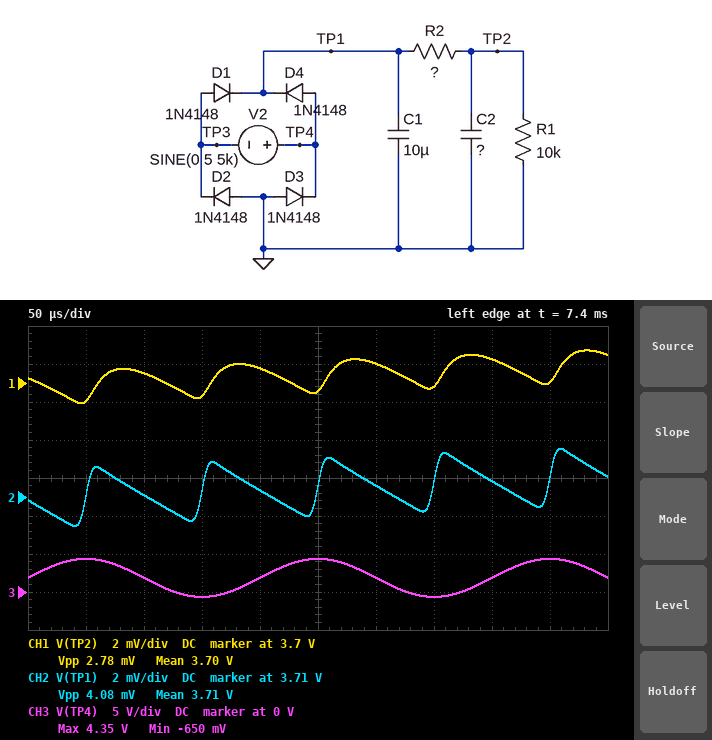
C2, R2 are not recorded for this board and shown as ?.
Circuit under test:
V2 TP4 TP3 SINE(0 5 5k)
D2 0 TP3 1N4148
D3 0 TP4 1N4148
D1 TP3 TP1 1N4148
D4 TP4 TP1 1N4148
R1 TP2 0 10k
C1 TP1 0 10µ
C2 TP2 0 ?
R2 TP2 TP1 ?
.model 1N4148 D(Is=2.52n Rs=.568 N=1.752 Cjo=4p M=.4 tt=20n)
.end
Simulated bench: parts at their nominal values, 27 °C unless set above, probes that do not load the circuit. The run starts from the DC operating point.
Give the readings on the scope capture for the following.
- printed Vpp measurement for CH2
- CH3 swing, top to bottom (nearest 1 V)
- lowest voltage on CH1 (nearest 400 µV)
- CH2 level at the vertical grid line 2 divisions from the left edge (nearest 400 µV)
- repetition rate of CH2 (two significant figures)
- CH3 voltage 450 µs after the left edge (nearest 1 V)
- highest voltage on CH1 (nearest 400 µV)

4.08 mV
5 V
3.6988 V
3.7100 V
10 kHz
4 V
3.7016 V
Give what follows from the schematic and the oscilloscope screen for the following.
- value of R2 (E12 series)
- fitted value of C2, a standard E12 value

27 Ω
680 nF
